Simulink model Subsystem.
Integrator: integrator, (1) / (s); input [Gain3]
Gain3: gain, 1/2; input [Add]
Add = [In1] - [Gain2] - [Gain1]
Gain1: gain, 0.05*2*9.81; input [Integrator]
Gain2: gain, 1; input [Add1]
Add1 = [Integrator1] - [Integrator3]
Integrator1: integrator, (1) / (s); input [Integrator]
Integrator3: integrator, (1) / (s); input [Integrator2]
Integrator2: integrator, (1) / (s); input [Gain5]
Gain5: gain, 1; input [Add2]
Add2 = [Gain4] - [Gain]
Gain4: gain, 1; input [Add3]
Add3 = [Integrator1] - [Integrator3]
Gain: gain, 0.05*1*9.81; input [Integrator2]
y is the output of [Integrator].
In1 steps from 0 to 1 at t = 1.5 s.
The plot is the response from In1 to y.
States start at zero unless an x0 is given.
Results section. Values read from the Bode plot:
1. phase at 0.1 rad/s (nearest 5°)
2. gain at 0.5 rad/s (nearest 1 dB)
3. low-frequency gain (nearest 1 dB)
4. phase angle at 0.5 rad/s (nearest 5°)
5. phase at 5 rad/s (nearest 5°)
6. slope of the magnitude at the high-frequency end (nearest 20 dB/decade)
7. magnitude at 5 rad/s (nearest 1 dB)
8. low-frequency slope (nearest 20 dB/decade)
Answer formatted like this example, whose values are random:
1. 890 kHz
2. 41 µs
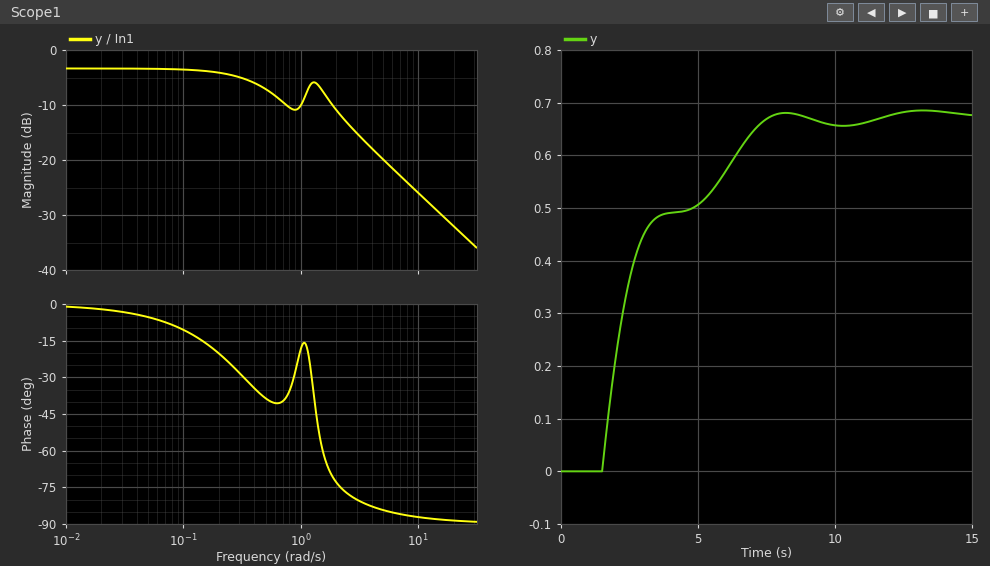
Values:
1. -10°
2. -7 dB
3. -3 dB
4. -40°
5. -85°
6. -20 dB/decade
7. -20 dB
8. 0 dB/decade
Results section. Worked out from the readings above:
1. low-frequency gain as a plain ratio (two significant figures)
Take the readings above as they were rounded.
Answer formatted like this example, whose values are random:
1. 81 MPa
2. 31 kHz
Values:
1. 0.71
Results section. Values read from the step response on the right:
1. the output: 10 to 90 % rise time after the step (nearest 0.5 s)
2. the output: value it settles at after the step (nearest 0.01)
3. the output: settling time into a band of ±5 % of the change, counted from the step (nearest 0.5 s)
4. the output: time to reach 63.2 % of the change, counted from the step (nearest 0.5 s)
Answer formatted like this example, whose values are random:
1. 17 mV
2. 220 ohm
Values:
1. 5.0 s
2. 0.68
3. 5.5 s
4. 1.5 s
